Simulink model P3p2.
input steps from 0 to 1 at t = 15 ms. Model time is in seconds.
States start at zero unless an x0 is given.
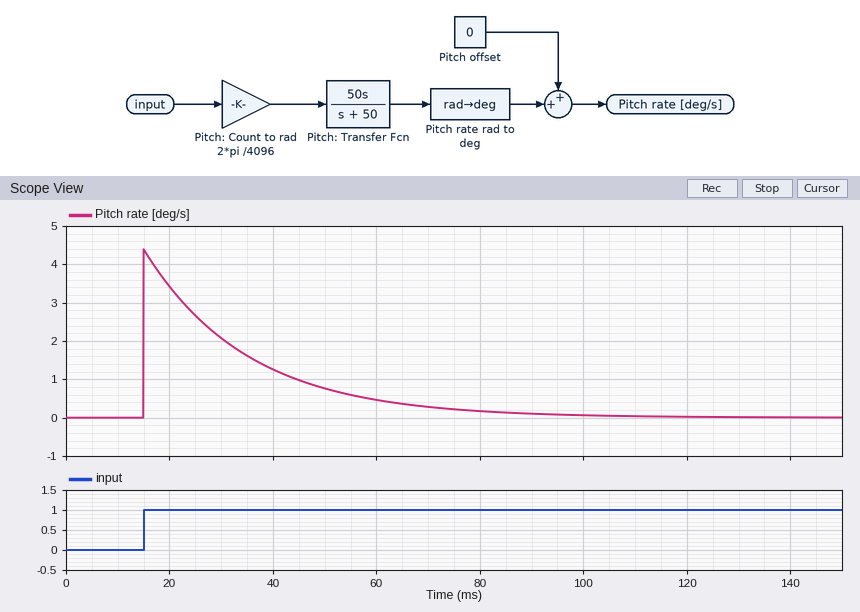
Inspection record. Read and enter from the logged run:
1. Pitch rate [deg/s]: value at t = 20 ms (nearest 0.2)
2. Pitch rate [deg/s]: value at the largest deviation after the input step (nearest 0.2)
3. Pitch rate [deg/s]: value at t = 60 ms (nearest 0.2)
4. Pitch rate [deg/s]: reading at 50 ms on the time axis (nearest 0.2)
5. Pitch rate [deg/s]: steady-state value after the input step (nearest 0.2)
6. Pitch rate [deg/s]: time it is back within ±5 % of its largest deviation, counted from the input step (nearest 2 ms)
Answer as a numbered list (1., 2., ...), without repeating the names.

1. 3.4
2. 4.4
3. 0.4
4. 0.8
5. 0.0
6. 60 ms
